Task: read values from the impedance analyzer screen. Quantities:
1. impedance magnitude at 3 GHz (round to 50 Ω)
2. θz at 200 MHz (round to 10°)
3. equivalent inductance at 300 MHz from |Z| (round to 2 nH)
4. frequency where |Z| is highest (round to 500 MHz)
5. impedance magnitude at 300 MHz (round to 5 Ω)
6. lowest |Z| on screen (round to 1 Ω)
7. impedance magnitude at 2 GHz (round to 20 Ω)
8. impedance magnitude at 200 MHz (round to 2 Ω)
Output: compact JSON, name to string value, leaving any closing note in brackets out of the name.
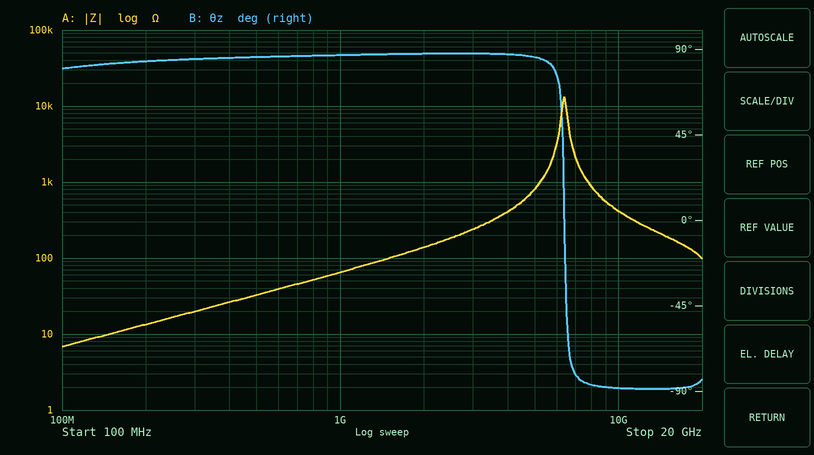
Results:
{"impedance magnitude at 3 GHz": "250 Ω", "θz at 200 MHz": "80°", "equivalent inductance at 300 MHz from |Z|": "10 nH", "frequency where |Z| is highest": "6.5 GHz", "impedance magnitude at 300 MHz": "20 Ω", "lowest |Z| on screen": "7 Ω", "impedance magnitude at 2 GHz": "140 Ω", "impedance magnitude at 200 MHz": "14 Ω"}
